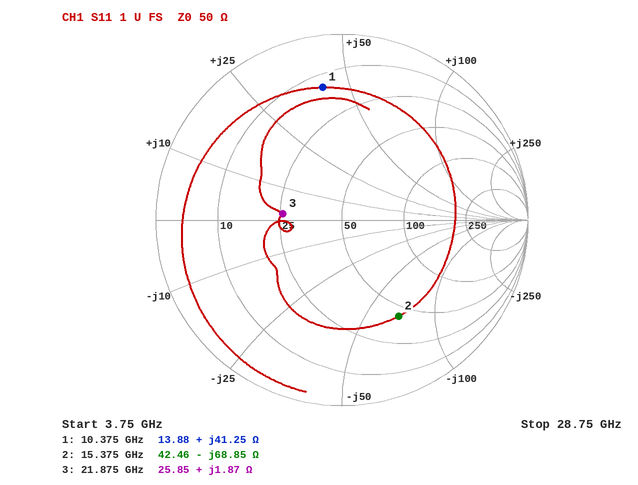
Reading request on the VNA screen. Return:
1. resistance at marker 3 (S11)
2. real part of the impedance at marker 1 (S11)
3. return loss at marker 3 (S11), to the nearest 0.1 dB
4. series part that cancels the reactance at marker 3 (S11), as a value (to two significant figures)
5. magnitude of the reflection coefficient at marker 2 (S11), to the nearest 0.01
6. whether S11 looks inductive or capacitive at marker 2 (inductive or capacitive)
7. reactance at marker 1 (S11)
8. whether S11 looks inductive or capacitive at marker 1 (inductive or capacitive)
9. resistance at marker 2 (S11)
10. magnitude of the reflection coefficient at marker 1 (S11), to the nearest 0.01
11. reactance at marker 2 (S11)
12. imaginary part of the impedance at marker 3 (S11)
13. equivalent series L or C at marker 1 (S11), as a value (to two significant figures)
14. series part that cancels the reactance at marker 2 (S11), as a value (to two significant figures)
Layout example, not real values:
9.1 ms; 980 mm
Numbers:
25.85 Ω; 13.88 Ω; 9.9 dB; 3.9 pF; 0.60; capacitive; +41.25 Ω; inductive; 42.46 Ω; 0.72; -68.85 Ω; +1.87 Ω; 630 pH; 710 pH
